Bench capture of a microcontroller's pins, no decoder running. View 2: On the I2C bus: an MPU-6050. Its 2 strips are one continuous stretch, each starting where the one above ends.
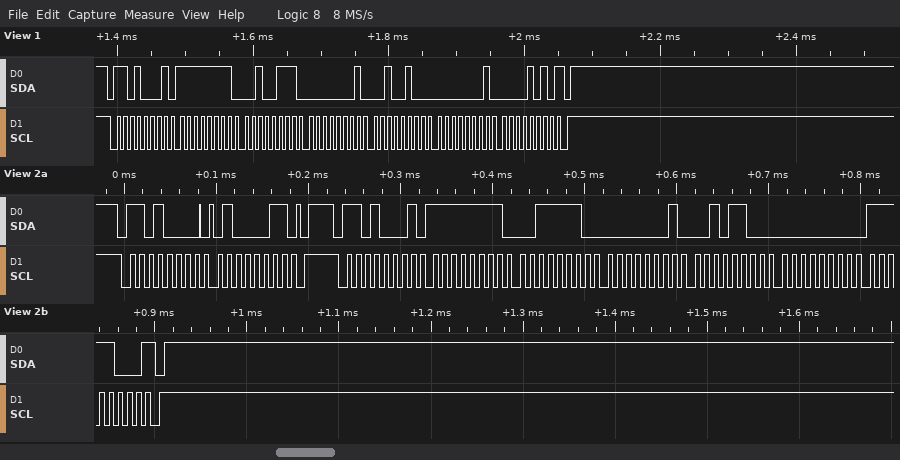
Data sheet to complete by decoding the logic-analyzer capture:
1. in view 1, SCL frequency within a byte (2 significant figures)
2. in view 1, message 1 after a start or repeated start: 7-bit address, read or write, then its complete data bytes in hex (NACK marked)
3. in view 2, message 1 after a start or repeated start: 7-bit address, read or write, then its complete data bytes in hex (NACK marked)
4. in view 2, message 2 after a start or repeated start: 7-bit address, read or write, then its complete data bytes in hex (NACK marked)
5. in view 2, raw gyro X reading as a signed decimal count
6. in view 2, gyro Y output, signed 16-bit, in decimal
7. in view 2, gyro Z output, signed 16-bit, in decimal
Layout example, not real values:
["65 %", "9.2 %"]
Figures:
["100 kHz", "0x68 read: FF 27 01 24 01 0A NACK", "0x68 write: 43", "0x68 read: FF 3E 01 2C 00 F8 NACK", "-194", "300", "248"]
